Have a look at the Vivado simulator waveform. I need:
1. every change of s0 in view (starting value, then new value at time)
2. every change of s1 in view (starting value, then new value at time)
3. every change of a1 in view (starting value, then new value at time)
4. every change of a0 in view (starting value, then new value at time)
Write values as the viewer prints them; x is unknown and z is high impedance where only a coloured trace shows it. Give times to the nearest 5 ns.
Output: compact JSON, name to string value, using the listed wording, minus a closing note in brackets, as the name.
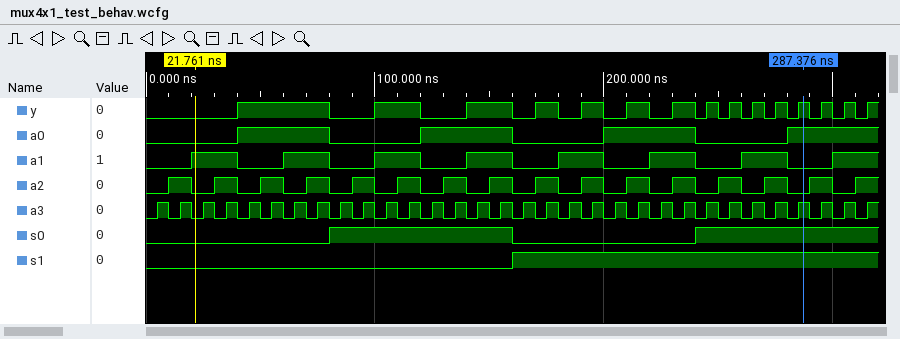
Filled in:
{"every change of s0 in view": "0, 1 at 80 ns, 0 at 160 ns, 1 at 240 ns", "every change of s1 in view": "0, 1 at 160 ns", "every change of a1 in view": "0, 1 at 20 ns, 0 at 40 ns, 1 at 60 ns, 0 at 80 ns, 1 at 100 ns, 0 at 120 ns, 1 at 140 ns, 0 at 160 ns, 1 at 180 ns, 0 at 200 ns, 1 at 220 ns, 0 at 240 ns, 1 at 260 ns, 0 at 280 ns, 1 at 300 ns", "every change of a0 in view": "0, 1 at 40 ns, 0 at 80 ns, 1 at 120 ns, 0 at 160 ns, 1 at 200 ns, 0 at 240 ns, 1 at 280 ns"}
